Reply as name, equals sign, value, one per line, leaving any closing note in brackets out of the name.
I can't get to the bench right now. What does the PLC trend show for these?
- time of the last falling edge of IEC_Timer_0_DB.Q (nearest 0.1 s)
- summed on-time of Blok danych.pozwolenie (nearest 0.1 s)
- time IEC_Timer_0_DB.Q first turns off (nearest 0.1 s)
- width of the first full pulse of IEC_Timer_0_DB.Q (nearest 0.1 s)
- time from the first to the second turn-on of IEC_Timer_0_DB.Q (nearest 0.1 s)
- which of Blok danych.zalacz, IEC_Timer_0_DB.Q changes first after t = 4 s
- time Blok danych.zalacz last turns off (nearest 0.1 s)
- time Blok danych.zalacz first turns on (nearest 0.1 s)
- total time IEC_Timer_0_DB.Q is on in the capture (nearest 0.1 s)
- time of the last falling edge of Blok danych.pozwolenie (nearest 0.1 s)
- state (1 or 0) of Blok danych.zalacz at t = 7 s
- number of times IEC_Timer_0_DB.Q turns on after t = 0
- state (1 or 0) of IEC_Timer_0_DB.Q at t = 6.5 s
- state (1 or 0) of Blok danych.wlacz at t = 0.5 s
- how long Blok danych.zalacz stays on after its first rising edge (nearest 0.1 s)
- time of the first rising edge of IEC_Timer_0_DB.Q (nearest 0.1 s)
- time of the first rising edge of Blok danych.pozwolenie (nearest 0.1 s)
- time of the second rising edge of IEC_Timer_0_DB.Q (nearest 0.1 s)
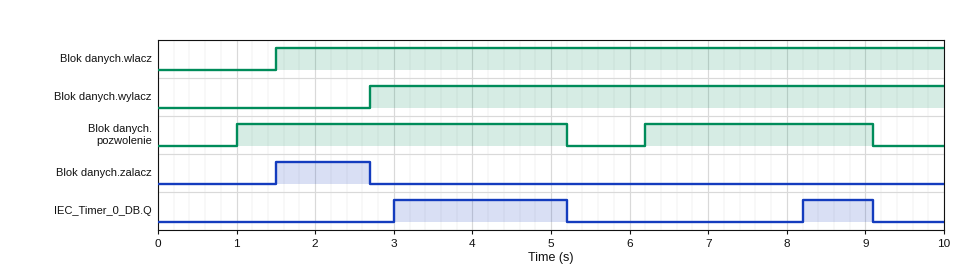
time of the last falling edge of IEC_Timer_0_DB.Q = 9.1 s
summed on-time of Blok danych.pozwolenie = 7.1 s
time IEC_Timer_0_DB.Q first turns off = 5.2 s
width of the first full pulse of IEC_Timer_0_DB.Q = 2.2 s
time from the first to the second turn-on of IEC_Timer_0_DB.Q = 5.2 s
which of Blok danych.zalacz, IEC_Timer_0_DB.Q changes first after t = 4 s = IEC_Timer_0_DB.Q
time Blok danych.zalacz last turns off = 2.7 s
time Blok danych.zalacz first turns on = 1.5 s
total time IEC_Timer_0_DB.Q is on in the capture = 3.1 s
time of the last falling edge of Blok danych.pozwolenie = 9.1 s
state (1 or 0) of Blok danych.zalacz at t = 7 s = 0
number of times IEC_Timer_0_DB.Q turns on after t = 0 = 2
state (1 or 0) of IEC_Timer_0_DB.Q at t = 6.5 s = 0
state (1 or 0) of Blok danych.wlacz at t = 0.5 s = 0
how long Blok danych.zalacz stays on after its first rising edge = 1.2 s
time of the first rising edge of IEC_Timer_0_DB.Q = 3.0 s
time of the first rising edge of Blok danych.pozwolenie = 1.0 s
time of the second rising edge of IEC_Timer_0_DB.Q = 8.2 s
